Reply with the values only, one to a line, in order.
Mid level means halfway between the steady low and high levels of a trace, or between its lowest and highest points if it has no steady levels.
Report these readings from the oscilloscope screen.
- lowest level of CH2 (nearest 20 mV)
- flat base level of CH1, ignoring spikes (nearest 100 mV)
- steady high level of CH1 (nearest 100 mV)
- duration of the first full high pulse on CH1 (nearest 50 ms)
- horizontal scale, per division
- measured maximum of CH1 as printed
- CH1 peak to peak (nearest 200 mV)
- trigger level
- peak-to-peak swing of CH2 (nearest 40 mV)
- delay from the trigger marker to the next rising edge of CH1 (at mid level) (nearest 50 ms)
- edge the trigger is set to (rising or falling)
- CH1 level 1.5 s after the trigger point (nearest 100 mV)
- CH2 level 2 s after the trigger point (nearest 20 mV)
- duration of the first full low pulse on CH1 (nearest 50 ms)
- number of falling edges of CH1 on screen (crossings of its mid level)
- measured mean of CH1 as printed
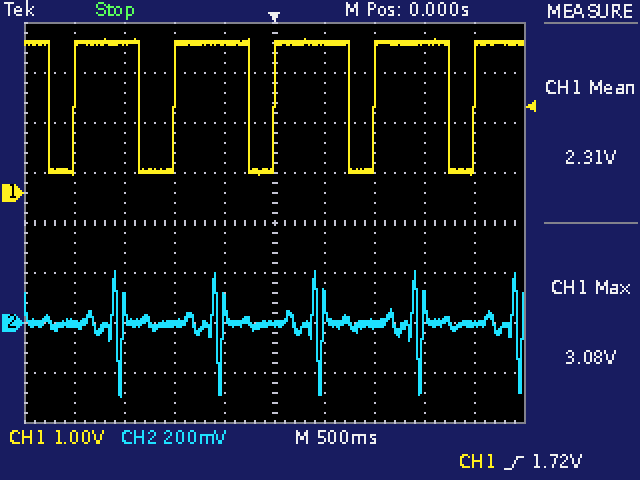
-300 mV
400 mV
3.0 V
650 ms
500 ms
3.08 V
2.8 V
1.72 V
520 mV
1.00 s
rising
3.0 V
0 mV
250 ms
5
2.31 V
